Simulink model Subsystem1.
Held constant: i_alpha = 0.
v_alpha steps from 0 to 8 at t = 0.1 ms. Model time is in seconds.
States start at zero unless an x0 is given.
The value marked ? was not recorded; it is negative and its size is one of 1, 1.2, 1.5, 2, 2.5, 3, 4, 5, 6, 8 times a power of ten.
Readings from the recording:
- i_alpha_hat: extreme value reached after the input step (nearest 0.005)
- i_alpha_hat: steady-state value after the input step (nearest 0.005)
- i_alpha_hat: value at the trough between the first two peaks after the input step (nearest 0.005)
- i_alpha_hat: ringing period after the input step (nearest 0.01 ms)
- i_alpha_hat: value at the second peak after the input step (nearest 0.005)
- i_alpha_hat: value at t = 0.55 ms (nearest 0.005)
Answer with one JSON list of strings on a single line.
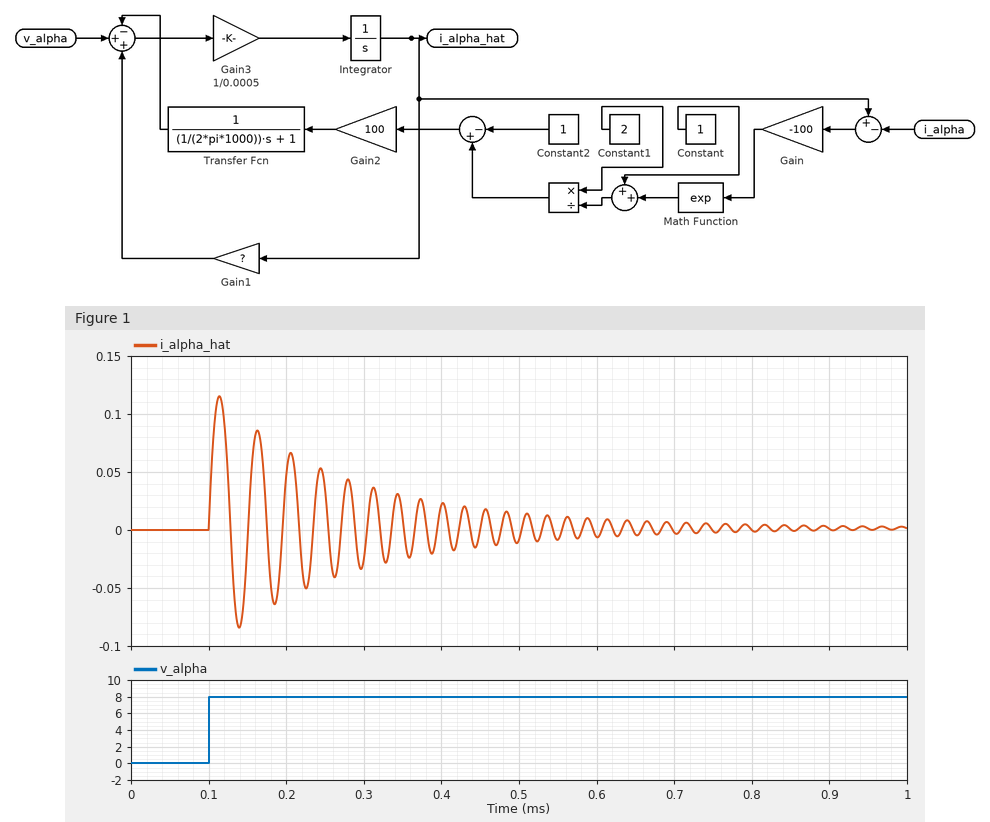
["0.115", "0.000", "-0.085", "0.05 ms", "0.085", "-0.010"]
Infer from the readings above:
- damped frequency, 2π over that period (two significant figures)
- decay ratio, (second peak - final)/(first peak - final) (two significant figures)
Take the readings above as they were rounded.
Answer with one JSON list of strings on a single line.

["130 rad/ms", "0.74"]
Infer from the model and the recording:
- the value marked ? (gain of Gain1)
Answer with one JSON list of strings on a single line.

["-1.5"]
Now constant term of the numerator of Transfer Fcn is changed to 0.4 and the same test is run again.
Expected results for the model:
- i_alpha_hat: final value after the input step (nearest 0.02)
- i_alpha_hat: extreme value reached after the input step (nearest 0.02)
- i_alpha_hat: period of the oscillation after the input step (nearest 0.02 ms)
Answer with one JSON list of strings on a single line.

["0.00", "0.26", "0.10 ms"]
